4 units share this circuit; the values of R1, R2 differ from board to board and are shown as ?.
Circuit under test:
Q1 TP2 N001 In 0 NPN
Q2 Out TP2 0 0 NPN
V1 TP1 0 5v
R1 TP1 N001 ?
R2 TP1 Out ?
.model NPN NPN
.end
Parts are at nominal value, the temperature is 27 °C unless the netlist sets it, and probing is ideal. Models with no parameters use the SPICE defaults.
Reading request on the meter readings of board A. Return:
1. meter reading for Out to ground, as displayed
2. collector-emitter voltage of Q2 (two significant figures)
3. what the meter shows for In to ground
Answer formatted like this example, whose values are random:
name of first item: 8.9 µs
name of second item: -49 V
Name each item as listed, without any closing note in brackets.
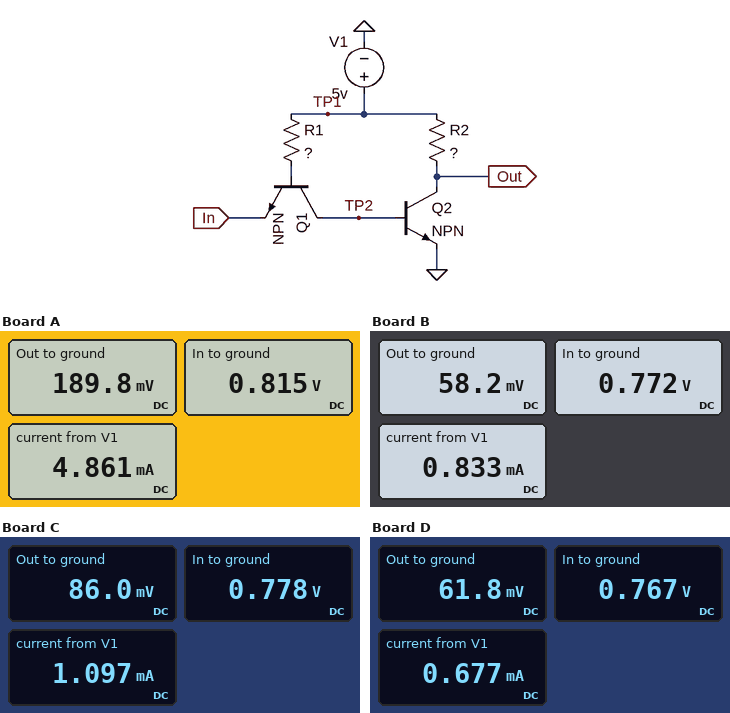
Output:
meter reading for Out to ground, as displayed: 189.8 mV
collector-emitter voltage of Q2: 190 mV
what the meter shows for In to ground: 0.815 V
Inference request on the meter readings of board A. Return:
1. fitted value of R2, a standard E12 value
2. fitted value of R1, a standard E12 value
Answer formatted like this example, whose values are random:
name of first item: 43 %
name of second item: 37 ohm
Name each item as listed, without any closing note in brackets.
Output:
fitted value of R2, a standard E12 value: 1 kΩ
fitted value of R1, a standard E12 value: 68 kΩ
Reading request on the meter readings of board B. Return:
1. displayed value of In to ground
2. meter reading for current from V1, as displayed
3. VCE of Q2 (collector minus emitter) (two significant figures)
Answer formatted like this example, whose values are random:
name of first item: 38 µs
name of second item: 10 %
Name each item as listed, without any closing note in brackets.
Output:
displayed value of In to ground: 0.772 V
meter reading for current from V1, as displayed: 0.833 mA
VCE of Q2 (collector minus emitter): 58 mV
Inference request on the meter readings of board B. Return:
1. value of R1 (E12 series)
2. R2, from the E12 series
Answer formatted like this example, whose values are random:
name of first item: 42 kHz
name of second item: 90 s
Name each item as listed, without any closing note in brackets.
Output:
value of R1: 33 kΩ
R2, from the E12 series: 6.8 kΩ
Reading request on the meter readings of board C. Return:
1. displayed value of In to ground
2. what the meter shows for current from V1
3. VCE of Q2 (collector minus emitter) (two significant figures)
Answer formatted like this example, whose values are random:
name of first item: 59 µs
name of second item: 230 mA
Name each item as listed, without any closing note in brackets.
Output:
displayed value of In to ground: 0.778 V
what the meter shows for current from V1: 1.097 mA
VCE of Q2 (collector minus emitter): 86 mV
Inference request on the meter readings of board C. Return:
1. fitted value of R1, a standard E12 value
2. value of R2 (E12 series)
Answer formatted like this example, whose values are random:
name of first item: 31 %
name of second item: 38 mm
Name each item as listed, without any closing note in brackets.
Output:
fitted value of R1, a standard E12 value: 68 kΩ
value of R2: 4.7 kΩ
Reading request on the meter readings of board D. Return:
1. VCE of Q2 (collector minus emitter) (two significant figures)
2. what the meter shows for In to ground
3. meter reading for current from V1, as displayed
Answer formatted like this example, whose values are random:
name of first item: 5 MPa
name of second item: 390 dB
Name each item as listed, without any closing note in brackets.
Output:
VCE of Q2 (collector minus emitter): 62 mV
what the meter shows for In to ground: 0.767 V
meter reading for current from V1, as displayed: 0.677 mA
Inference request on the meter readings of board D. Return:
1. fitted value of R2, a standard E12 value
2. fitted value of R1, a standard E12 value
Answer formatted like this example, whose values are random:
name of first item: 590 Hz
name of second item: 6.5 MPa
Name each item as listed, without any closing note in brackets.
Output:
fitted value of R2, a standard E12 value: 8.2 kΩ
fitted value of R1, a standard E12 value: 47 kΩ
